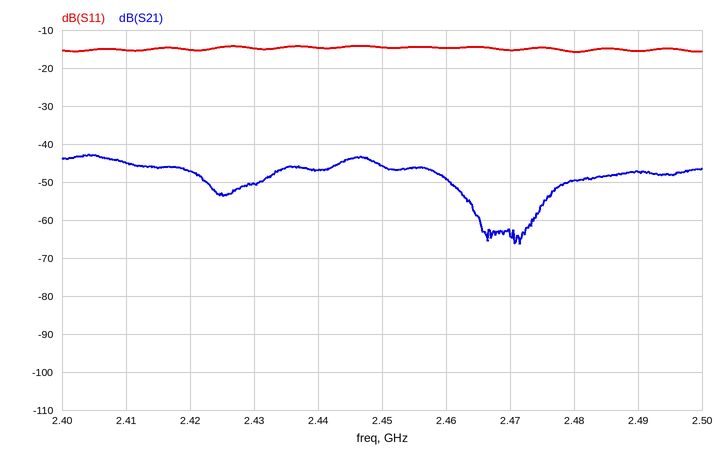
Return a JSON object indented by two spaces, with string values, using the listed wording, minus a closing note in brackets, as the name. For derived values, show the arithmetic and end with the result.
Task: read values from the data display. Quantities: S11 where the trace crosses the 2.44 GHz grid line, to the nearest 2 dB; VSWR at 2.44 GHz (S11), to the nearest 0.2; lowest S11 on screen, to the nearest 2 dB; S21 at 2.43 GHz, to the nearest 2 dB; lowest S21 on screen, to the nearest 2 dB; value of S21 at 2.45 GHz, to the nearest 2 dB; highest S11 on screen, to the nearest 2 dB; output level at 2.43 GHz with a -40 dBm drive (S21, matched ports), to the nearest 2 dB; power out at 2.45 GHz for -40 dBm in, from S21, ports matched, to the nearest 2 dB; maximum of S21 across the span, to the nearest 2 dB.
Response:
{
  "S11 where the trace crosses the 2.44 GHz grid line, to the nearest 2 dB": "-14 dB",
  "VSWR at 2.44 GHz (S11), to the nearest 0.2": "|Γ| = 10^(-14/20) = 0.1995; VSWR = (1 + 0.1995)/(1 − 0.1995) ≈ 1.50, so 1.4 to the nearest 0.2",
  "lowest S11 on screen, to the nearest 2 dB": "-16 dB",
  "S21 at 2.43 GHz, to the nearest 2 dB": "-50 dB",
  "lowest S21 on screen, to the nearest 2 dB": "-66 dB",
  "value of S21 at 2.45 GHz, to the nearest 2 dB": "-46 dB",
  "highest S11 on screen, to the nearest 2 dB": "-14 dB",
  "output level at 2.43 GHz with a -40 dBm drive (S21, matched ports), to the nearest 2 dB": "-40 dBm + (-50 dB) = -90 dBm",
  "power out at 2.45 GHz for -40 dBm in, from S21, ports matched, to the nearest 2 dB": "-40 dBm + (-46 dB) = -86 dBm",
  "maximum of S21 across the span, to the nearest 2 dB": "-42 dB"
}
